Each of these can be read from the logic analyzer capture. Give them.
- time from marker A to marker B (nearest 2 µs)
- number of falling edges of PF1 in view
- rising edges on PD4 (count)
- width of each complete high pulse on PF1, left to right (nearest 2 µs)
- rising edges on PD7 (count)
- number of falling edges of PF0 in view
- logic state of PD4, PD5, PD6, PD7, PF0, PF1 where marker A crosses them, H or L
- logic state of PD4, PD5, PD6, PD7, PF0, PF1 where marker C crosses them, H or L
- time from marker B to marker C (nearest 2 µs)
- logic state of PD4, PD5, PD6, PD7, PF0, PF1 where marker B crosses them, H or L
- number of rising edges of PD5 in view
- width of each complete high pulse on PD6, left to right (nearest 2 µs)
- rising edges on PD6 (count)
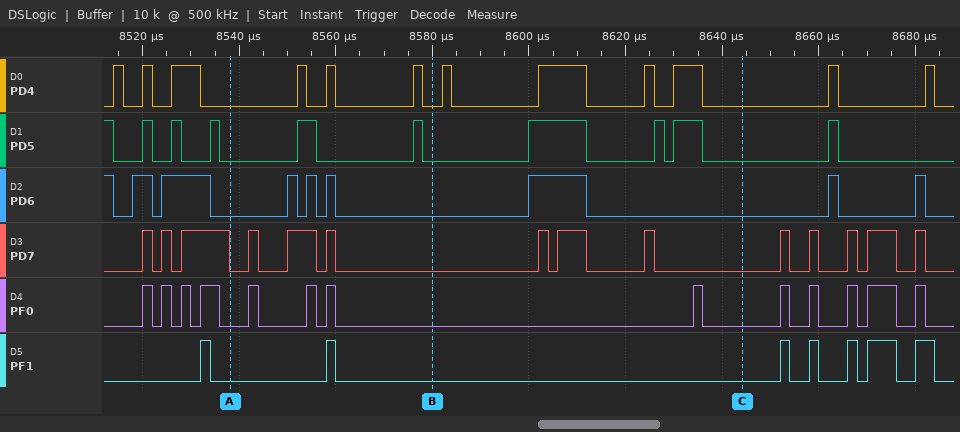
42 µs
7
12
2 µs, 2 µs, 2 µs, 2 µs, 2 µs, 6 µs, 4 µs
14
13
PD4=L, PD5=L, PD6=L, PD7=L, PF0=L, PF1=L
PD4=L, PD5=L, PD6=L, PD7=L, PF0=L, PF1=L
64 µs
PD4=L, PD5=L, PD6=L, PD7=L, PF0=L, PF1=L
9
4 µs, 10 µs, 2 µs, 2 µs, 2 µs, 12 µs, 2 µs, 2 µs
8
